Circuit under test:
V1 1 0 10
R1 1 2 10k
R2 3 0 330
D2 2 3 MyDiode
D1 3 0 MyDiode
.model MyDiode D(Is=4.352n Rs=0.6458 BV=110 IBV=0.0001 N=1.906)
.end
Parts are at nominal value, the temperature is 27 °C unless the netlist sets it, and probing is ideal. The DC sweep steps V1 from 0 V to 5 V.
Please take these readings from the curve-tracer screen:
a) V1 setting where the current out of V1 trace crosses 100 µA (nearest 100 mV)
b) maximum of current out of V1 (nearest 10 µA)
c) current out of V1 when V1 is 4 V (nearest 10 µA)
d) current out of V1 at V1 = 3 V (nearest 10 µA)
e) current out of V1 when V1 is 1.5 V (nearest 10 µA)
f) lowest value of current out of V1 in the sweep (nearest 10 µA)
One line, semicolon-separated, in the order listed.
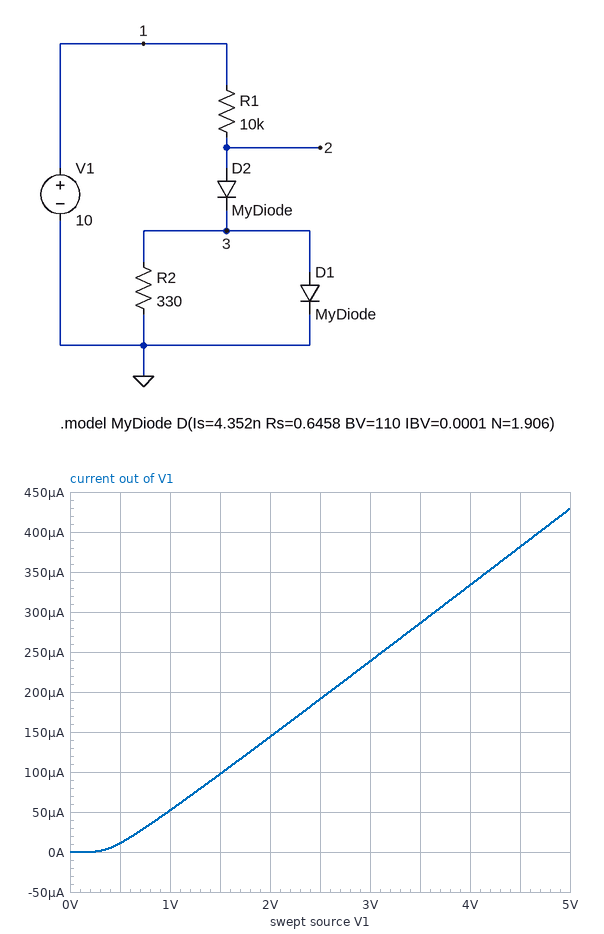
1.5 V; 430 µA; 330 µA; 240 µA; 100 µA; 0 A
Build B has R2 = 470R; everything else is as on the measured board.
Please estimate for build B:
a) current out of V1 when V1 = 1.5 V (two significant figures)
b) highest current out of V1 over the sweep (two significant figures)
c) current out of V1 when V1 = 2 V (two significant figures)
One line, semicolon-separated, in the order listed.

96 µA; 420 µA; 140 µA
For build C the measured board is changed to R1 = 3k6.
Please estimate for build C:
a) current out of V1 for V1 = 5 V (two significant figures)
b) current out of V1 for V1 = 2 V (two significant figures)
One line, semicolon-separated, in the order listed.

1.1 mA; 370 µA
